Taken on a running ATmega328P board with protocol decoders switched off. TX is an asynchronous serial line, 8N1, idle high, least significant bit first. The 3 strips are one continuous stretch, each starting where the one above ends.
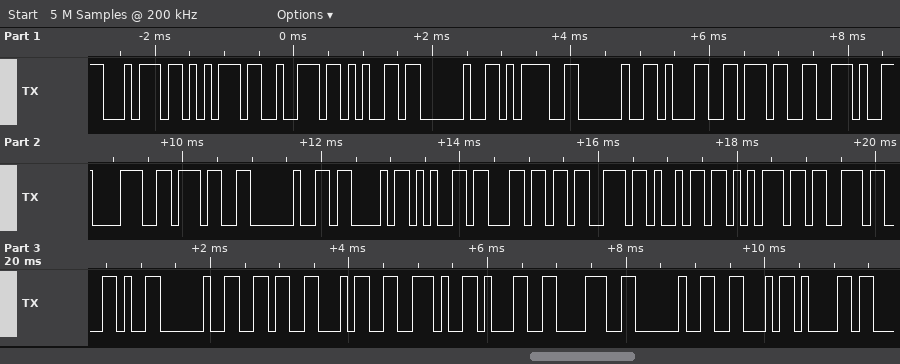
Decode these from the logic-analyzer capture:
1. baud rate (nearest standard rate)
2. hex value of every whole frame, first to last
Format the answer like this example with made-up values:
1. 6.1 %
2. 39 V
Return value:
1. 9600 baud
2. 74 75 72 65 20 3D 20 31 37 2E 38 37 20 43 65 6C 73 69 75 73 2C 20 36 34 2E 31 38 20 46 61
